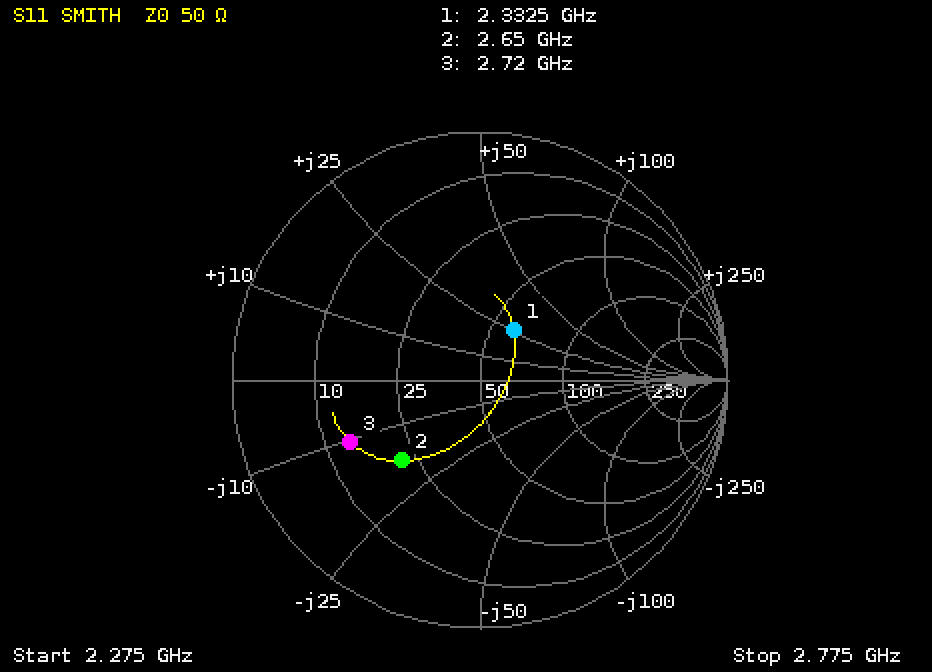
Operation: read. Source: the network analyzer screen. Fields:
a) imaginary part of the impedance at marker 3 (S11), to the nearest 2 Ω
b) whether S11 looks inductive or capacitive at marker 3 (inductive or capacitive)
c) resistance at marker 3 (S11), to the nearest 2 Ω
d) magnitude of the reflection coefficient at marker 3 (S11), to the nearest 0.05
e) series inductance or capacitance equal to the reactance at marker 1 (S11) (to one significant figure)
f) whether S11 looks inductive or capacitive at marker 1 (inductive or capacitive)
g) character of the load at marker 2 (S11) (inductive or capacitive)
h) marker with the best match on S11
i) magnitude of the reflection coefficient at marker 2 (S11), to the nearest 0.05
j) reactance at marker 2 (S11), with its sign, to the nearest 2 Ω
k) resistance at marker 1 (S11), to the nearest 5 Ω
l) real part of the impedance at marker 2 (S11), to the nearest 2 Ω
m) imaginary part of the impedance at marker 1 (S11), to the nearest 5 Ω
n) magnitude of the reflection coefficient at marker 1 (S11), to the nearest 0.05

-10 Ω
capacitive
14 Ω
0.60
2 nH
inductive
capacitive
marker 1
0.45
-18 Ω
60 Ω
22 Ω
+25 Ω
0.25
